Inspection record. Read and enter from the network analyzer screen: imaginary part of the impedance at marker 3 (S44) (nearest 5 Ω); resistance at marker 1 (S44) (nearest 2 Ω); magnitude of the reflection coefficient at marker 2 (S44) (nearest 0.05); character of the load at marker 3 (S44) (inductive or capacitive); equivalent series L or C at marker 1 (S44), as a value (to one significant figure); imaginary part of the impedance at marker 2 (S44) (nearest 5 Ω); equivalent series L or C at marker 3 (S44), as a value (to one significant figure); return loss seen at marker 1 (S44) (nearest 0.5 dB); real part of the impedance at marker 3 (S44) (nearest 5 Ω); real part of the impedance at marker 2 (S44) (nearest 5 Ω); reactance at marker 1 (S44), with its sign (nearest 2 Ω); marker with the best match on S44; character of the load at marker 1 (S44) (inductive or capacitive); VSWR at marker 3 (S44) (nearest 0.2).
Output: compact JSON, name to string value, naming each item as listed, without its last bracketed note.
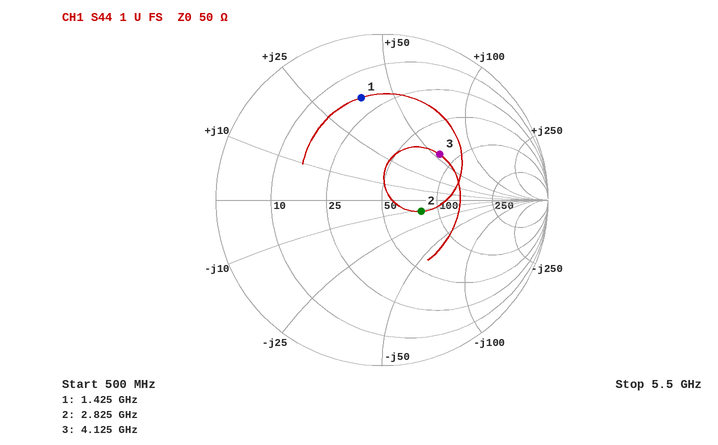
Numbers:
{"imaginary part of the impedance at marker 3 (S44)": "+55 Ω", "resistance at marker 1 (S44)": "18 Ω", "magnitude of the reflection coefficient at marker 2 (S44)": "0.25", "character of the load at marker 3 (S44)": "inductive", "equivalent series L or C at marker 1 (S44), as a value": "4 nH", "imaginary part of the impedance at marker 2 (S44)": "-10 Ω", "equivalent series L or C at marker 3 (S44), as a value": "2 nH", "return loss seen at marker 1 (S44)": "4.0 dB", "real part of the impedance at marker 3 (S44)": "80 Ω", "real part of the impedance at marker 2 (S44)": "80 Ω", "reactance at marker 1 (S44), with its sign": "+38 Ω", "marker with the best match on S44": "marker 2", "character of the load at marker 1 (S44)": "inductive", "VSWR at marker 3 (S44)": "2.6"}
